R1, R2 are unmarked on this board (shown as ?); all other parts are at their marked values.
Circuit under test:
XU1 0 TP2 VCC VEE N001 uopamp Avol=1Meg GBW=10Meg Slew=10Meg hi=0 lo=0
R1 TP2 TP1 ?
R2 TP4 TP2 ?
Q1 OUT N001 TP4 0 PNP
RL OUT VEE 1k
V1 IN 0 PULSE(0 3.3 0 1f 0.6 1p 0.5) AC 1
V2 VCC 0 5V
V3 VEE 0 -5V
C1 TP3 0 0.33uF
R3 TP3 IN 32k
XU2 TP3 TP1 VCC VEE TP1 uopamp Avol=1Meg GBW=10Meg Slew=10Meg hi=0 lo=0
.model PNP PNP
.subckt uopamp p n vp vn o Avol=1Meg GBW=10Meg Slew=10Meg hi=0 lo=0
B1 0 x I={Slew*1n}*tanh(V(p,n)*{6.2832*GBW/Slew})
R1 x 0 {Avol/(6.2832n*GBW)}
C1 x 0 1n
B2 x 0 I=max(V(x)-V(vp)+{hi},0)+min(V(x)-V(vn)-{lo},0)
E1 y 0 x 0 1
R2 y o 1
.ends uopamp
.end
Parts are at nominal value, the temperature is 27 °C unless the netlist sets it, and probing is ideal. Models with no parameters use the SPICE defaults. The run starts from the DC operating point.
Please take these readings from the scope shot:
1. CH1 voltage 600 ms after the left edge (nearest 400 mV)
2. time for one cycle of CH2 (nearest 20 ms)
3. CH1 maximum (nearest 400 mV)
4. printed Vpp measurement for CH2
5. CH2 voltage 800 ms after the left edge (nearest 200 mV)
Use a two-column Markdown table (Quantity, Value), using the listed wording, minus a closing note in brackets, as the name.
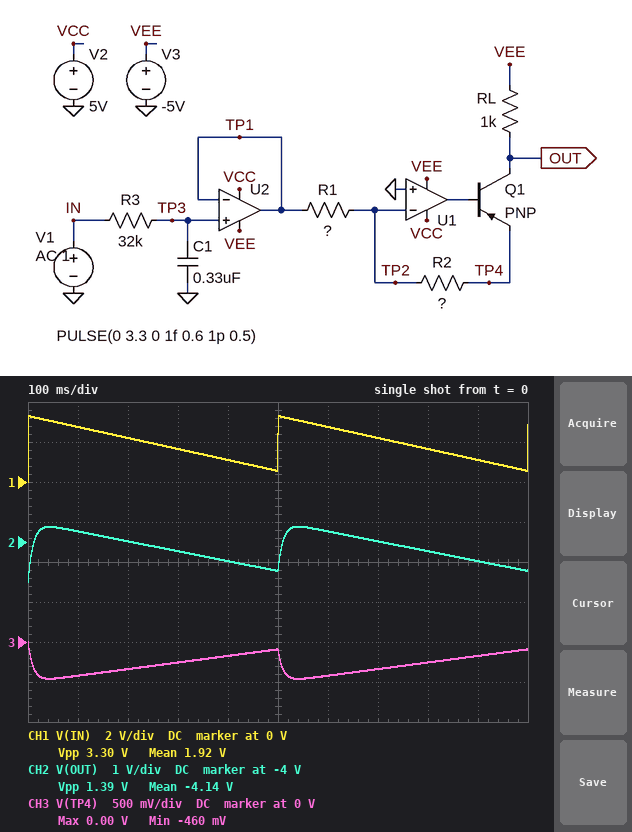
| Quantity | Value |
|---|---|
| CH1 voltage 600 ms after the left edge | 2.8 V |
| time for one cycle of CH2 | 500 ms |
| CH1 maximum | 3.2 V |
| printed Vpp measurement for CH2 | 1.39 V |
| CH2 voltage 800 ms after the left edge | -4.2 V |
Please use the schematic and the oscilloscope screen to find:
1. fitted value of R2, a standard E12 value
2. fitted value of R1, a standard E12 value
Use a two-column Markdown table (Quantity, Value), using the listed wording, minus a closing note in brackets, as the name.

| Quantity | Value |
|---|---|
| fitted value of R2, a standard E12 value | 330 Ω |
| fitted value of R1, a standard E12 value | 2.2 kΩ |
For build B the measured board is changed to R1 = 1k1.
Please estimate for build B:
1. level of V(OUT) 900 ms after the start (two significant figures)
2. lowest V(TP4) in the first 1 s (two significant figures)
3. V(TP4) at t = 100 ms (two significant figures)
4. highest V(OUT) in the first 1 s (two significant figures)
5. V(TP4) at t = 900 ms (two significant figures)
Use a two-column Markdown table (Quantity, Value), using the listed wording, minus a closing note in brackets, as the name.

| Quantity | Value |
|---|---|
| level of V(OUT) 900 ms after the start | -4.0 V |
| lowest V(TP4) in the first 1 s | -920 mV |
| V(TP4) at t = 100 ms | -840 mV |
| highest V(OUT) in the first 1 s | -2.2 V |
| V(TP4) at t = 900 ms | -350 mV |
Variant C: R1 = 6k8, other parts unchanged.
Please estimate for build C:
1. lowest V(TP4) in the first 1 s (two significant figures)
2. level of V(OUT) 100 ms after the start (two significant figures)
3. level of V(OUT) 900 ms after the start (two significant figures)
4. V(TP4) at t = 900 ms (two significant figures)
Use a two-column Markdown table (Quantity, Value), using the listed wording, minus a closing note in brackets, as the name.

| Quantity | Value |
|---|---|
| lowest V(TP4) in the first 1 s | -150 mV |
| level of V(OUT) 100 ms after the start | -4.6 V |
| level of V(OUT) 900 ms after the start | -4.8 V |
| V(TP4) at t = 900 ms | -56 mV |
